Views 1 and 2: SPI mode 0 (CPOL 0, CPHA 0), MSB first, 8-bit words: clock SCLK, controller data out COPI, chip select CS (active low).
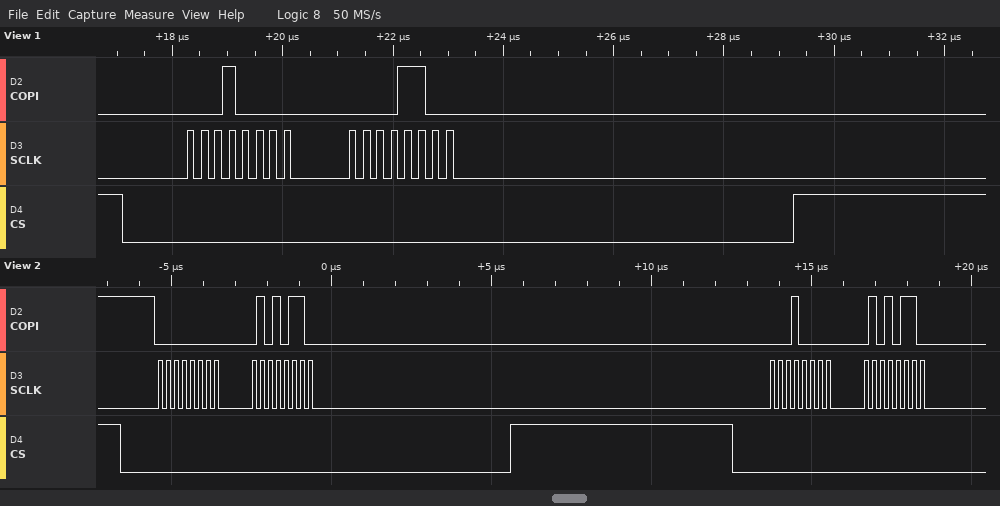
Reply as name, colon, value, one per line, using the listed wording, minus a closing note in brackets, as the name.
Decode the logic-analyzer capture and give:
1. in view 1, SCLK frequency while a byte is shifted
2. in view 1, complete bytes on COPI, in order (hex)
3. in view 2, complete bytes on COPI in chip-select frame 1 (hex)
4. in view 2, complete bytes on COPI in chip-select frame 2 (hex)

in view 1, SCLK frequency while a byte is shifted: 4 MHz
in view 1, complete bytes on COPI, in order: 10 0C
in view 2, complete bytes on COPI in chip-select frame 1: 00 56
in view 2, complete bytes on COPI in chip-select frame 2: 10 56
